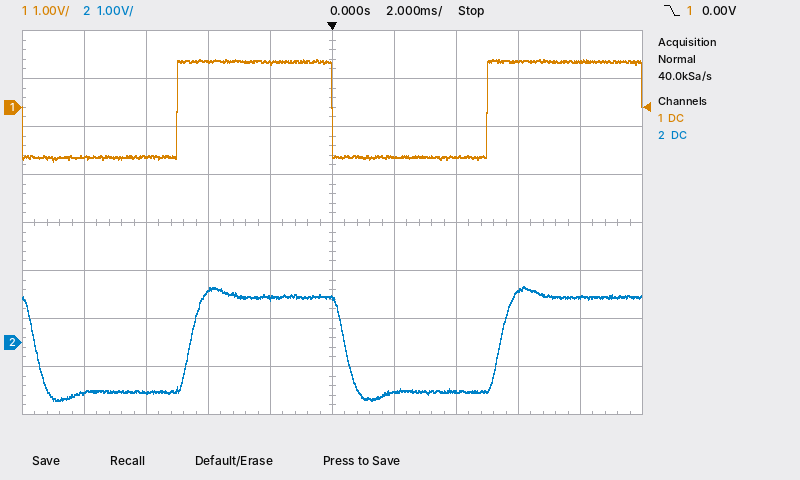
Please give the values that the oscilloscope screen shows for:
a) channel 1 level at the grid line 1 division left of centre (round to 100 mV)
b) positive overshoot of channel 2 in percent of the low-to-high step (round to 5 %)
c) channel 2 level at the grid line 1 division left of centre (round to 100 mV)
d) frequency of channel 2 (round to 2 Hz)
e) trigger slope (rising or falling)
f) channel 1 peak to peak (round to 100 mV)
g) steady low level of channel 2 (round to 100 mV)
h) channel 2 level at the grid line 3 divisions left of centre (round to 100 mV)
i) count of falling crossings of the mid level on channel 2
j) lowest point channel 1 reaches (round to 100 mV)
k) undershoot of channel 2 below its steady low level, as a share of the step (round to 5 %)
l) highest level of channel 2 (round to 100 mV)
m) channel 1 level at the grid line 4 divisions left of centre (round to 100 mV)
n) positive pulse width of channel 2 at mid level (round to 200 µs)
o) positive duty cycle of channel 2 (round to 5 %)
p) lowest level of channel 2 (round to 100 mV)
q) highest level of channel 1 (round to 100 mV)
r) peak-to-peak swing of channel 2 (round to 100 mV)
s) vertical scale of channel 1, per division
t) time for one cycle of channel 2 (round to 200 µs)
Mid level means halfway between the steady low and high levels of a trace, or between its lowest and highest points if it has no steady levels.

900 mV
10 %
900 mV
100 Hz
falling
2.1 V
-1.0 V
-1.0 V
2
-1.1 V
10 %
1.2 V
-1.0 V
5.0 ms
50 %
-1.2 V
1.0 V
2.4 V
1 V
10.0 ms
